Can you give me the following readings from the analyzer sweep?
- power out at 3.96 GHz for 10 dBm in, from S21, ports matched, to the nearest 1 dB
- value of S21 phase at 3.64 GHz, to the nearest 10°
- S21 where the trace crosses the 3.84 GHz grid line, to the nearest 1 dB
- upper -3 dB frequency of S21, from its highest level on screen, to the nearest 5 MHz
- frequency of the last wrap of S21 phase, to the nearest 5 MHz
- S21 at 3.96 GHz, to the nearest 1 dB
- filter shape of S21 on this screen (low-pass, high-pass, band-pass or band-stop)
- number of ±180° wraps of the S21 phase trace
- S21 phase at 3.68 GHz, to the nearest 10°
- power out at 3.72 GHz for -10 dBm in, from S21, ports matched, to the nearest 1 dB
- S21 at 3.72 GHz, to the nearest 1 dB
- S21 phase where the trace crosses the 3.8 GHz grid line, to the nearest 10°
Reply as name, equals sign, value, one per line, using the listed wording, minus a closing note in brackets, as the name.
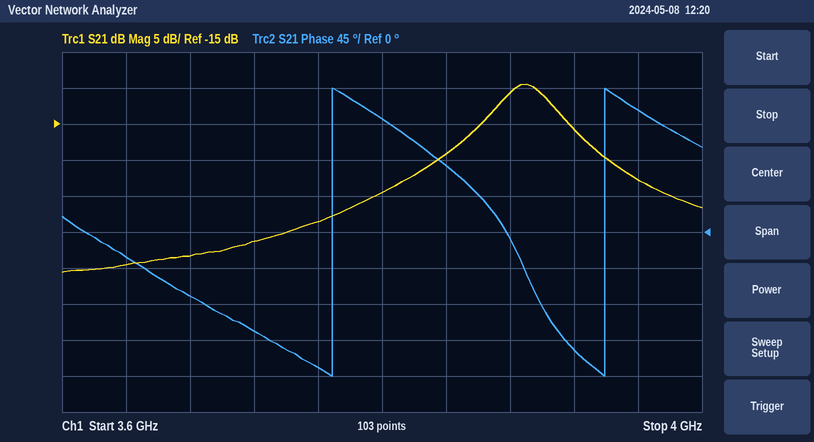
power out at 3.96 GHz for 10 dBm in, from S21, ports matched, to the nearest 1 dB = -13 dBm
value of S21 phase at 3.64 GHz, to the nearest 10° = -30°
S21 where the trace crosses the 3.84 GHz grid line, to the nearest 1 dB = -19 dB
upper -3 dB frequency of S21, from its highest level on screen, to the nearest 5 MHz = 3.905 GHz
frequency of the last wrap of S21 phase, to the nearest 5 MHz = 3.940 GHz
S21 at 3.96 GHz, to the nearest 1 dB = -23 dB
filter shape of S21 on this screen = band-pass
number of ±180° wraps of the S21 phase trace = 2
S21 phase at 3.68 GHz, to the nearest 10° = -80°
power out at 3.72 GHz for -10 dBm in, from S21, ports matched, to the nearest 1 dB = -41 dBm
S21 at 3.72 GHz, to the nearest 1 dB = -31 dB
S21 phase where the trace crosses the 3.8 GHz grid line, to the nearest 10° = 140°
